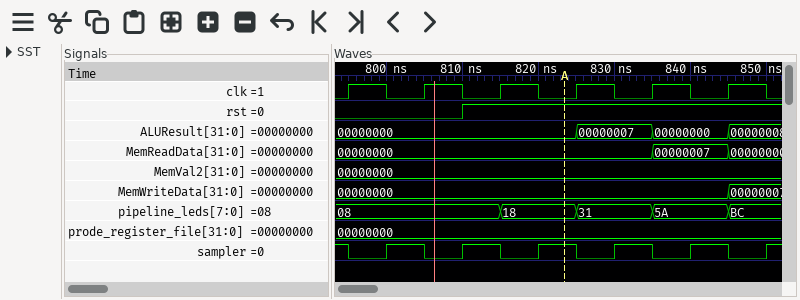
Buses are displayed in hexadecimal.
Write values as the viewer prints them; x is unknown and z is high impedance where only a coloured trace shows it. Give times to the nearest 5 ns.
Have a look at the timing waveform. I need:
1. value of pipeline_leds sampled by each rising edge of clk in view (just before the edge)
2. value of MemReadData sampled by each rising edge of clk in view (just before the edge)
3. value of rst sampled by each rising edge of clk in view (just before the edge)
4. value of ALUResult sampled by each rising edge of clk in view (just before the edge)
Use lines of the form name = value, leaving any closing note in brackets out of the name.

value of pipeline_leds sampled by each rising edge of clk in view = 08, 08, 08, 18, 31, 5A
value of MemReadData sampled by each rising edge of clk in view = 00000000, 00000000, 00000000, 00000000, 00000000, 00000007
value of rst sampled by each rising edge of clk in view = 0 0 1 1 1 1
value of ALUResult sampled by each rising edge of clk in view = 00000000, 00000000, 00000000, 00000000, 00000007, 00000000
